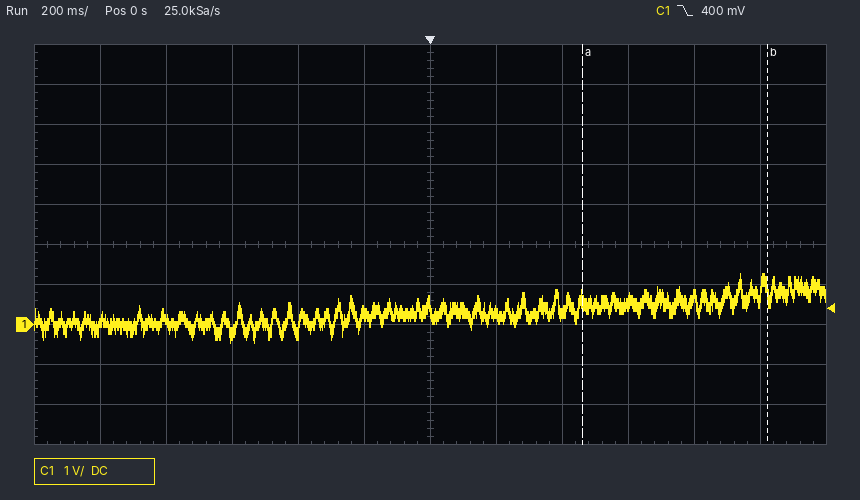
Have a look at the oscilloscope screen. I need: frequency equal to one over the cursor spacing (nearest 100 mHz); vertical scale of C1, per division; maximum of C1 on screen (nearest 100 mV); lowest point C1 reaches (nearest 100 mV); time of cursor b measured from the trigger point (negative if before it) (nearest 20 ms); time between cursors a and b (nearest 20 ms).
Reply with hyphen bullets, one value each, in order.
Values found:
- 1.8 Hz
- 1 V
- 1.3 V
- -500 mV
- +1.02 s
- 560 ms
